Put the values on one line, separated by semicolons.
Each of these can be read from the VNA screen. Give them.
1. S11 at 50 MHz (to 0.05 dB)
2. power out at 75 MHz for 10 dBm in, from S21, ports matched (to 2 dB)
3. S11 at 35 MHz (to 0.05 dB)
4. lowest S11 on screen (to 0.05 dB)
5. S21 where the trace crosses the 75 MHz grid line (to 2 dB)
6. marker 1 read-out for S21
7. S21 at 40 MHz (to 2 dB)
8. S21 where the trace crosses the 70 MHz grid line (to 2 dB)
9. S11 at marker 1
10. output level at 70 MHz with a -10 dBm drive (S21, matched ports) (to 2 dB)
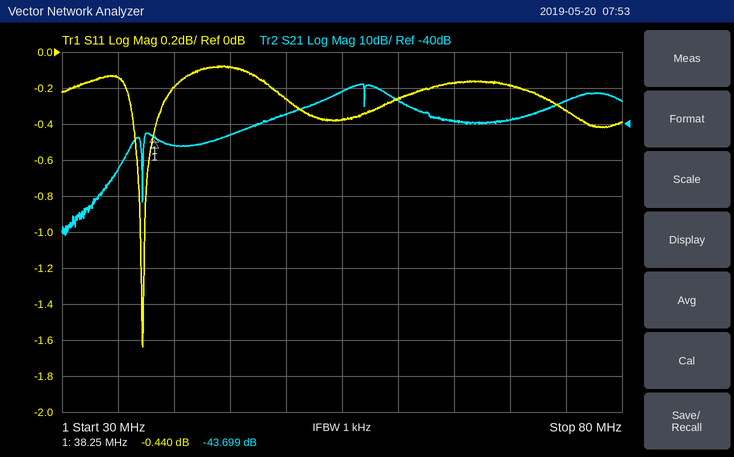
-0.25 dB; -24 dBm; -0.15 dB; -1.65 dB; -34 dB; -43.699 dB; -46 dB; -38 dB; -0.440 dB; -48 dBm
